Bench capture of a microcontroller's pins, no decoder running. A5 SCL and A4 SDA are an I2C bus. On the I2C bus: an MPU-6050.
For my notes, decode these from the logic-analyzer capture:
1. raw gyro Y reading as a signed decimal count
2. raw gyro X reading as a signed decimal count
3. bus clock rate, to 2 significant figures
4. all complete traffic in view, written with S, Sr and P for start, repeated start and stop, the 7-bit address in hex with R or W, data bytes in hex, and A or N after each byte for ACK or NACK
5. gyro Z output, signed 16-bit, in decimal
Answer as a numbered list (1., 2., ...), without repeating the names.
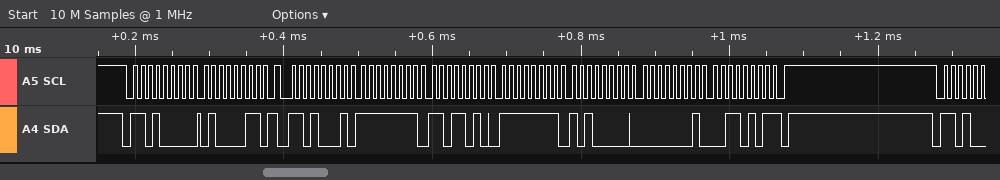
1. -96
2. -38
3. 100 kHz
4. S 68W A 43 A Sr 68R A FF A DA A FF A A0 A 01 A 35 N P
5. 309
